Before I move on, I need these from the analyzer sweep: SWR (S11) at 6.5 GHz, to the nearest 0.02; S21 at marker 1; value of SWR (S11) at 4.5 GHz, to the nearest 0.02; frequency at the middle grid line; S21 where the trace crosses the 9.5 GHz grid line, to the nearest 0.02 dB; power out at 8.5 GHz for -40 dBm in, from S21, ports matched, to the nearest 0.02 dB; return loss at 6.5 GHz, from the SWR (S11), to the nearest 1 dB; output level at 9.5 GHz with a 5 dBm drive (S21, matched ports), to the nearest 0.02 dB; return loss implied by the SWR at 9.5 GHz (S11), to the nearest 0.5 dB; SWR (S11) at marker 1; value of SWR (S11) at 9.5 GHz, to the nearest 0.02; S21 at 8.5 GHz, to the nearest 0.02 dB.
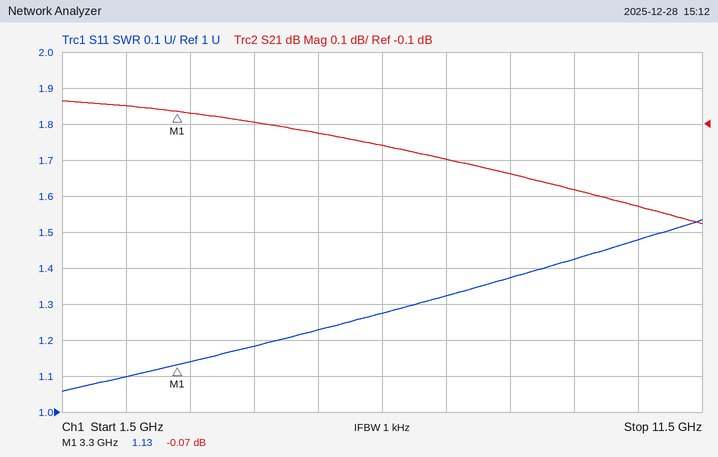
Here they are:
1.28
-0.07 dB
1.18
6.5 GHz
-0.28 dB
-40.24 dBm
18 dB
4.72 dBm
15.0 dB
1.13
1.42
-0.24 dB
